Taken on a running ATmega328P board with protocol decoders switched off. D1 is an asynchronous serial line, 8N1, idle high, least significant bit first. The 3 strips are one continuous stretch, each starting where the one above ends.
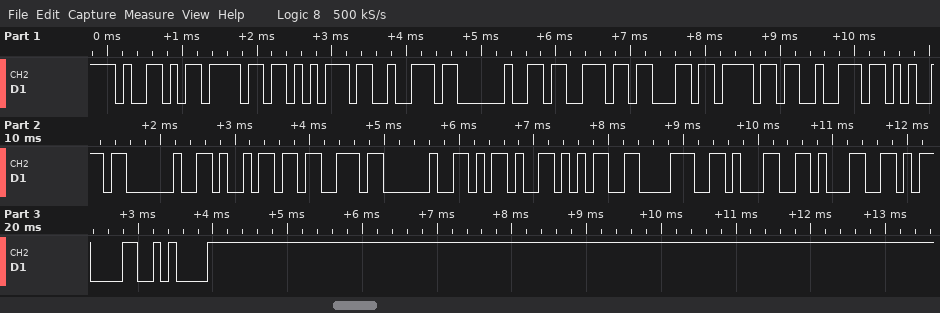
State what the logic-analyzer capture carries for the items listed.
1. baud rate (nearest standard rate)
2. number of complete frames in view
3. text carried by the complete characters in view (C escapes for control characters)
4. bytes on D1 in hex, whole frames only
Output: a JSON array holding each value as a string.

["9600 baud", "21", "\"Your score is -5811\\r\\n\"", "59 6F 75 72 20 73 63 6F 72 65 20 69 73 20 2D 35 38 31 31 0D 0A"]
